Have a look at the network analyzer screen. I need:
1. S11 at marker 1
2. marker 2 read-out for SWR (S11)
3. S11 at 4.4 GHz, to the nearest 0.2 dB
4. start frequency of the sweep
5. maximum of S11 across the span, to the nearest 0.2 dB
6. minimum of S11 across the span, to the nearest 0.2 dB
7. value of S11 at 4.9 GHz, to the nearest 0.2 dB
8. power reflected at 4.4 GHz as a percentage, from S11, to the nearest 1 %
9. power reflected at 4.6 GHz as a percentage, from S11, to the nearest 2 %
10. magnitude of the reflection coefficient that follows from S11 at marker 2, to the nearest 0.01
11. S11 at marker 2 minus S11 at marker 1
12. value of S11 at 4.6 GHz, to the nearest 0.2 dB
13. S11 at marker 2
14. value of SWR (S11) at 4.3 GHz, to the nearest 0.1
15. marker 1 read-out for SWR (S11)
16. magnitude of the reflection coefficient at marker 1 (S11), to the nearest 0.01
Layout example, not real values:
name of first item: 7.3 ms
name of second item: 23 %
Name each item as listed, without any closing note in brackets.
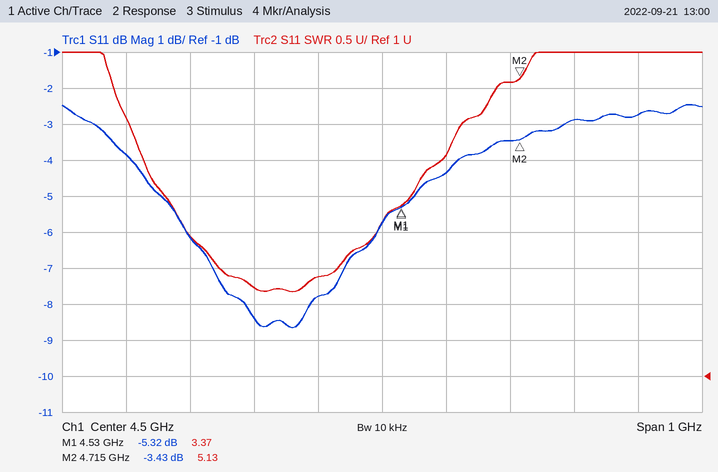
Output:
S11 at marker 1: -5.32 dB
marker 2 read-out for SWR: 5.13
S11 at 4.4 GHz, to the nearest 0.2 dB: -7.8 dB
start frequency of the sweep: 4 GHz
maximum of S11 across the span, to the nearest 0.2 dB: -2.4 dB
minimum of S11 across the span, to the nearest 0.2 dB: -8.6 dB
value of S11 at 4.9 GHz, to the nearest 0.2 dB: -2.8 dB
power reflected at 4.4 GHz as a percentage, from S11, to the nearest 1 %: 17 %
power reflected at 4.6 GHz as a percentage, from S11, to the nearest 2 %: 36 %
magnitude of the reflection coefficient that follows from S11 at marker 2, to the nearest 0.01: 0.67
S11 at marker 2 minus S11 at marker 1: 1.89 dB
value of S11 at 4.6 GHz, to the nearest 0.2 dB: -4.4 dB
S11 at marker 2: -3.43 dB
value of SWR (S11) at 4.3 GHz, to the nearest 0.1: 2.2
marker 1 read-out for SWR: 3.37
magnitude of the reflection coefficient at marker 1 (S11), to the nearest 0.01: 0.54
